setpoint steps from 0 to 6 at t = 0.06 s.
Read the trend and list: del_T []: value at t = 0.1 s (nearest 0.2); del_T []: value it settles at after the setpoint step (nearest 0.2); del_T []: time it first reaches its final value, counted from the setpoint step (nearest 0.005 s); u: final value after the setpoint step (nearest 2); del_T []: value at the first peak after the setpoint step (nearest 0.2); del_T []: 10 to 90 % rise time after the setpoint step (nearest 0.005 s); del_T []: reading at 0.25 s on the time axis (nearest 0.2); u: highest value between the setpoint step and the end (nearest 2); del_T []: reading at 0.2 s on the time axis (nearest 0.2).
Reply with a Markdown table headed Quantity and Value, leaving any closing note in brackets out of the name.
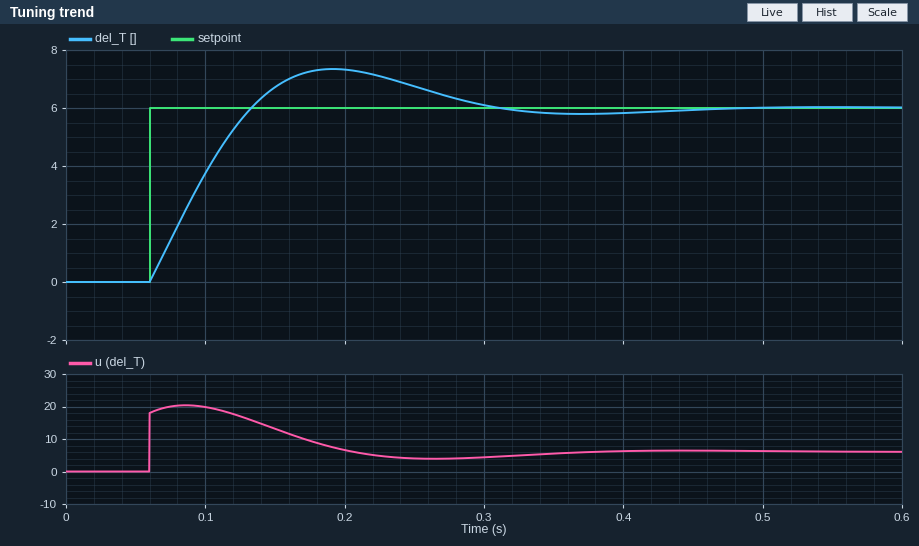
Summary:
| Quantity | Value |
|---|---|
| del_T []: value at t = 0.1 s | 3.8 |
| del_T []: value it settles at after the setpoint step | 6.0 |
| del_T []: time it first reaches its final value, counted from the setpoint step | 0.075 s |
| u: final value after the setpoint step | 6 |
| del_T []: value at the first peak after the setpoint step | 7.4 |
| del_T []: 10 to 90 % rise time after the setpoint step | 0.055 s |
| del_T []: reading at 0.25 s on the time axis | 6.8 |
| u: highest value between the setpoint step and the end | 20 |
| del_T []: reading at 0.2 s on the time axis | 7.4 |
